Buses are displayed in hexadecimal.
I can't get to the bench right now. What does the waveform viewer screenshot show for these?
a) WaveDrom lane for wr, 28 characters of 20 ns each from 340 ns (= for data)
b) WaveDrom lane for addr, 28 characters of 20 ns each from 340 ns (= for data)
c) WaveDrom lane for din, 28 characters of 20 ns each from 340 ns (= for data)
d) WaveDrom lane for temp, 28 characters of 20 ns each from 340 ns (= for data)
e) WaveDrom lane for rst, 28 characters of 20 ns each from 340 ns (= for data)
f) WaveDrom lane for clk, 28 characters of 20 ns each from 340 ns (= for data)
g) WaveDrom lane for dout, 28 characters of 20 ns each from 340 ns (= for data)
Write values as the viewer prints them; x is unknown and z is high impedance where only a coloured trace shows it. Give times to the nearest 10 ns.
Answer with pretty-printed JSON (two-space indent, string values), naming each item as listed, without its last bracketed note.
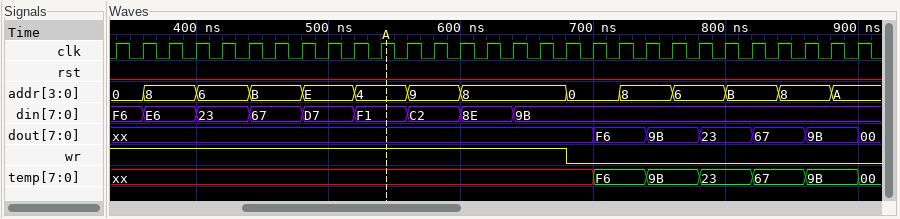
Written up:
{
  "WaveDrom lane for wr, 28 characters of 20 ns each from 340 ns": "{name: 'wr', wave: '1................0..........'}",
  "WaveDrom lane for addr, 28 characters of 20 ns each from 340 ns": "{name: 'addr', wave: '==.=.=.=.=.=.=...=.=.=.=.=.=', data: '0 8 6 B E 4 9 8 0 8 6 B 8 A'}",
  "WaveDrom lane for din, 28 characters of 20 ns each from 340 ns": "{name: 'din', wave: '==.=.=.=.=.=.=.=............', data: 'F6 E6 23 67 D7 F1 C2 8E 9B'}",
  "WaveDrom lane for temp, 28 characters of 20 ns each from 340 ns": "{name: 'temp', wave: 'x.................=.=.=.=.=.', data: 'F6 9B 23 67 9B'}",
  "WaveDrom lane for rst, 28 characters of 20 ns each from 340 ns": "{name: 'rst', wave: '0...........................'}",
  "WaveDrom lane for clk, 28 characters of 20 ns each from 340 ns": "{name: 'clk', wave: 'p...........................'}",
  "WaveDrom lane for dout, 28 characters of 20 ns each from 340 ns": "{name: 'dout', wave: 'x.................=.=.=.=.=.', data: 'F6 9B 23 67 9B'}"
}
